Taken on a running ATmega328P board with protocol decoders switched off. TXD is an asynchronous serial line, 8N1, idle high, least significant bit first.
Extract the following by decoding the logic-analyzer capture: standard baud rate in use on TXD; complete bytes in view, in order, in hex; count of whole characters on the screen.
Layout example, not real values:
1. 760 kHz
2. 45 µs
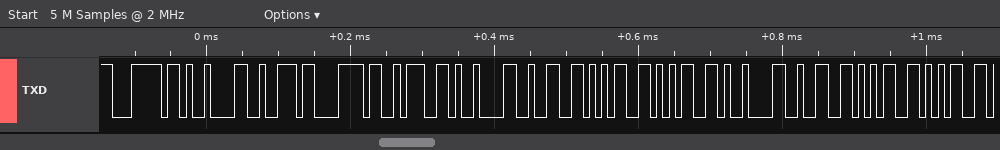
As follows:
1. 115200 baud
2. 0x7C 0x09 0x72 0x78 0x3A 0x09 0x32 0x35 0x35 0x09 0x32 0x35 0x35
3. 13
